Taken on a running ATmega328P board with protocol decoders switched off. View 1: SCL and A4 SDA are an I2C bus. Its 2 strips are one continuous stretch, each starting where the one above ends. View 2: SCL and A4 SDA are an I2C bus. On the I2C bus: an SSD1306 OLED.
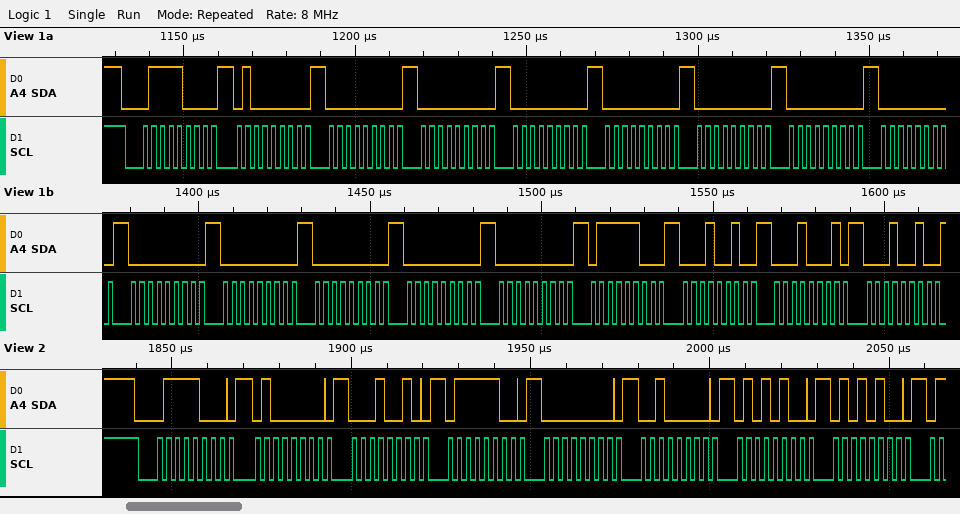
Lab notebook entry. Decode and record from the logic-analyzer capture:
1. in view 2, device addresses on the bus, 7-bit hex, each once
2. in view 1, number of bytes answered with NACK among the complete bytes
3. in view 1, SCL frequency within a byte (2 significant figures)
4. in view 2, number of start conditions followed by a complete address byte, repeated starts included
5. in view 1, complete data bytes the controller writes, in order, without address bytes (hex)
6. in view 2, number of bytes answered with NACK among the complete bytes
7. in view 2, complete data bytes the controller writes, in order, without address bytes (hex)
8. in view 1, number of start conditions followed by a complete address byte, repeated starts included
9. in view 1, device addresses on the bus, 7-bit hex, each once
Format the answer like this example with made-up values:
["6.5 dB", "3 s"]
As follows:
["0x3C", "0", "400 kHz", "1", "40 00 00 00 00 00 00 00 00 00 00 00 00 7C 12 11 12", "0", "40 12 7C 00 20 54 54", "1", "0x3C"]
